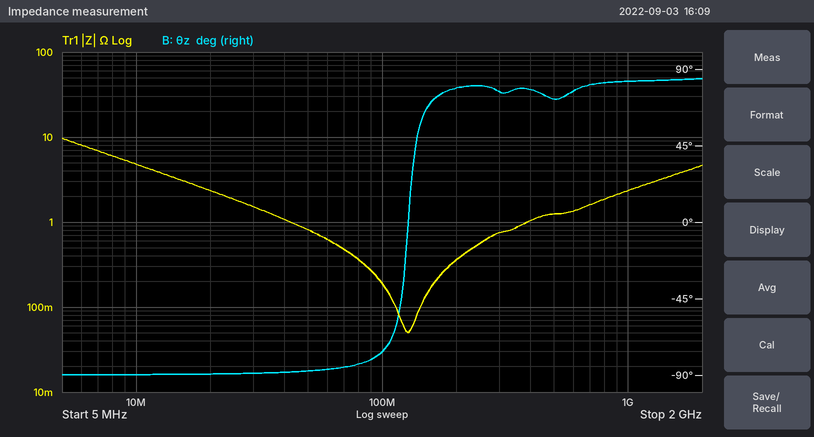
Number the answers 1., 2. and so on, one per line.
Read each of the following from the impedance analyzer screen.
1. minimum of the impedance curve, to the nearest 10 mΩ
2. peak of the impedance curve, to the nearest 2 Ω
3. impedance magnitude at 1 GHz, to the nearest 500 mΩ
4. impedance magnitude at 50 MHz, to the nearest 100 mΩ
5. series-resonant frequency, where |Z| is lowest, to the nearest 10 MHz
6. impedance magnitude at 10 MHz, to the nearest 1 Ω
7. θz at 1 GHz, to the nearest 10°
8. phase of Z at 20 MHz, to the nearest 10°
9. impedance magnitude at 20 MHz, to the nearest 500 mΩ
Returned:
1. 50 mΩ
2. 10 Ω
3. 2.5 Ω
4. 800 mΩ
5. 130 MHz
6. 5 Ω
7. 80°
8. -90°
9. 2.5 Ω
